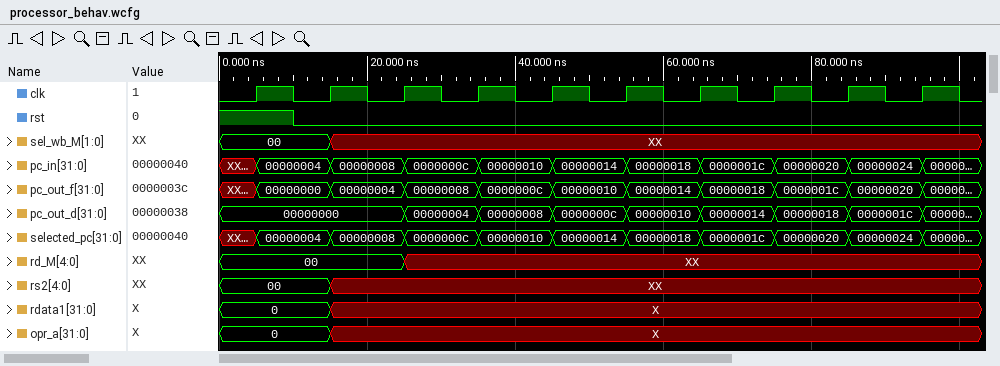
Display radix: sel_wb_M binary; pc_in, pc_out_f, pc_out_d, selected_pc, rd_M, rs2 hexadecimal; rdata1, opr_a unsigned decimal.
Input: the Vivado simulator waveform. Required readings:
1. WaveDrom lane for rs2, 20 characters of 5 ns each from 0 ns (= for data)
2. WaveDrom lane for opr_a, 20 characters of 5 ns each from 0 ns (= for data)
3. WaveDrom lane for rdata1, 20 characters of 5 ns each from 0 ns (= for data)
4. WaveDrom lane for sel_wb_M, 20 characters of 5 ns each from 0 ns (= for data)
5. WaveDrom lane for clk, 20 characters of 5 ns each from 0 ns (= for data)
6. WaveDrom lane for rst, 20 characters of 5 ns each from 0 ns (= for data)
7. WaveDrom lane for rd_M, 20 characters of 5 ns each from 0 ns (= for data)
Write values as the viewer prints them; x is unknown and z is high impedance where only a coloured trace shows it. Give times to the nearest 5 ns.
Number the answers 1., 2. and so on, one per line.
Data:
1. {name: 'rs2', wave: '=..x................', data: '00'}
2. {name: 'opr_a', wave: '=..x................', data: '0'}
3. {name: 'rdata1', wave: '=..x................', data: '0'}
4. {name: 'sel_wb_M', wave: '=..x................', data: '00'}
5. {name: 'clk', wave: '01010101010101010101'}
6. {name: 'rst', wave: '1.0.................'}
7. {name: 'rd_M', wave: '=....x..............', data: '00'}
